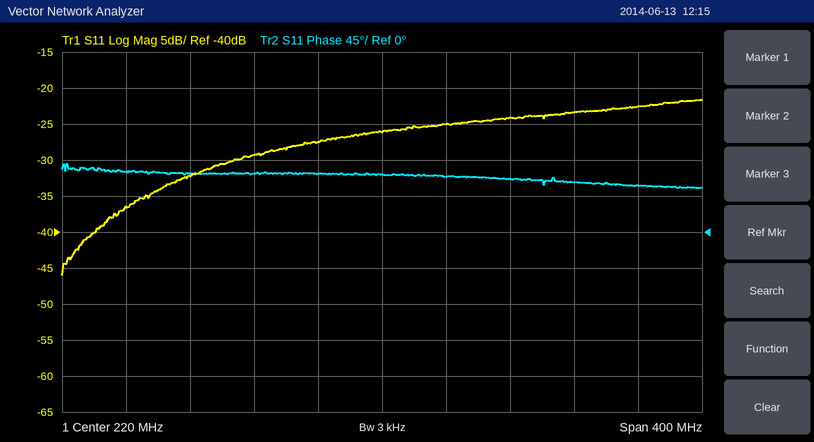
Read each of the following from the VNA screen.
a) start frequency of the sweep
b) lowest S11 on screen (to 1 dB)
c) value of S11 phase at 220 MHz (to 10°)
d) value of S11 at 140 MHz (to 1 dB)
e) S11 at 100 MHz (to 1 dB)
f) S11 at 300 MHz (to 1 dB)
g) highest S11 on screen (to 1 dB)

20 MHz
-46 dB
70°
-29 dB
-32 dB
-24 dB
-22 dB
